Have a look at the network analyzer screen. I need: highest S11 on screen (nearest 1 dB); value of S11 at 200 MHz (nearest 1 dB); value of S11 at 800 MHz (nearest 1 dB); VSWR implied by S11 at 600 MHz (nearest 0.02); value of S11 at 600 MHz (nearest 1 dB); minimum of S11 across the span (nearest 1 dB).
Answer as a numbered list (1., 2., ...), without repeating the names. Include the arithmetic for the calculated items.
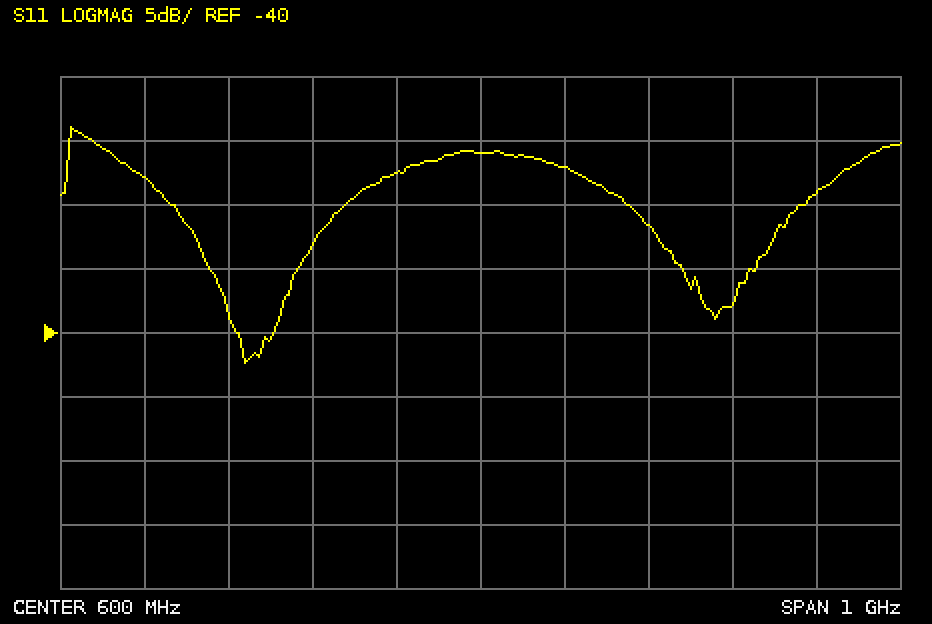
1. -24 dB
2. -28 dB
3. -32 dB
4. |Γ| = 10^(-26/20) = 0.0501; VSWR = (1 + 0.0501)/(1 − 0.0501) ≈ 1.11, so 1.10 to the nearest 0.02
5. -26 dB
6. -42 dB
